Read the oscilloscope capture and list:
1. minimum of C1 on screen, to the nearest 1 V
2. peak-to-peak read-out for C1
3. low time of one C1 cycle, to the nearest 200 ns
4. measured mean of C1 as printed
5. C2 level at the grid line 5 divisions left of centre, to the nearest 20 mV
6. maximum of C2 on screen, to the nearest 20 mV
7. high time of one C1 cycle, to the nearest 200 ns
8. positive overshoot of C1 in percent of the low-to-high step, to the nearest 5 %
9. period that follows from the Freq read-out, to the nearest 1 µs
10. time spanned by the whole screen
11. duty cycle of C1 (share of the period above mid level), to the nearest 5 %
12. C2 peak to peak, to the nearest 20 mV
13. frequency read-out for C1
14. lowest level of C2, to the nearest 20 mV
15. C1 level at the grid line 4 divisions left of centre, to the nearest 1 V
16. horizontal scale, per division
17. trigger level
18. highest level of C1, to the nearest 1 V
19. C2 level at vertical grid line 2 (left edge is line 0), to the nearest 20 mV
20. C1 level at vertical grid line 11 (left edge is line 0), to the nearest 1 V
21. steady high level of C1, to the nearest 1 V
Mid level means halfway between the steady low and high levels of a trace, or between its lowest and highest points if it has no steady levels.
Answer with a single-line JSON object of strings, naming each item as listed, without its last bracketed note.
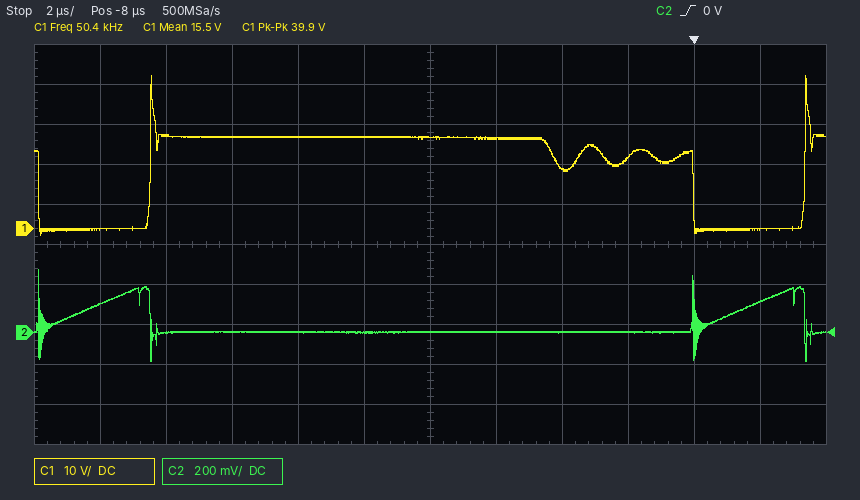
{"minimum of C1 on screen, to the nearest 1 V": "-2 V", "peak-to-peak read-out for C1": "39.9 V", "low time of one C1 cycle, to the nearest 200 ns": "3.4 µs", "measured mean of C1 as printed": "15.5 V", "C2 level at the grid line 5 divisions left of centre, to the nearest 20 mV": "140 mV", "maximum of C2 on screen, to the nearest 20 mV": "320 mV", "high time of one C1 cycle, to the nearest 200 ns": "16.4 µs", "positive overshoot of C1 in percent of the low-to-high step, to the nearest 5 %": "65 %", "period that follows from the Freq read-out, to the nearest 1 µs": "20 µs", "time spanned by the whole screen": "24 µs", "duty cycle of C1 (share of the period above mid level), to the nearest 5 %": "85 %", "C2 peak to peak, to the nearest 20 mV": "460 mV", "frequency read-out for C1": "50.4 kHz", "lowest level of C2, to the nearest 20 mV": "-140 mV", "C1 level at the grid line 4 divisions left of centre, to the nearest 1 V": "23 V", "horizontal scale, per division": "2 µs", "trigger level": "0 V", "highest level of C1, to the nearest 1 V": "38 V", "C2 level at vertical grid line 2 (left edge is line 0), to the nearest 20 mV": "0 mV", "C1 level at vertical grid line 11 (left edge is line 0), to the nearest 1 V": "0 V", "steady high level of C1, to the nearest 1 V": "23 V"}
